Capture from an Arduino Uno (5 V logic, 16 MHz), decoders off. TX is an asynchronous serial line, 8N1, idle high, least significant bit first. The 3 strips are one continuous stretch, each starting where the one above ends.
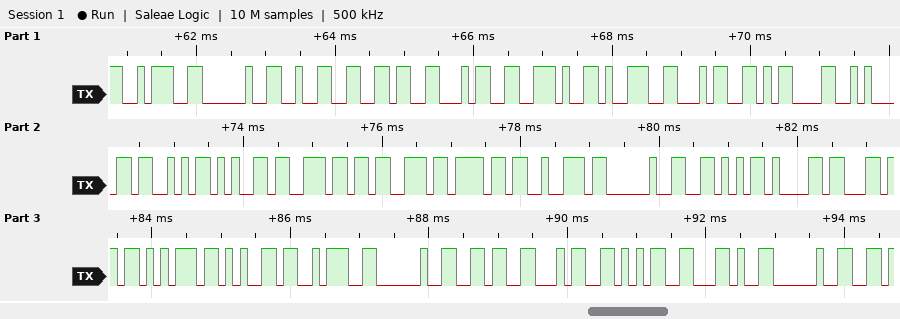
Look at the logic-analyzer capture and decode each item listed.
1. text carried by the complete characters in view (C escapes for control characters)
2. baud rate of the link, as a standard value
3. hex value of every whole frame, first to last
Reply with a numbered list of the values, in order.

1. ": 264.94\r\nSensor Value: 645, "
2. 9600 baud
3. 0x3A 0x20 0x32 0x36 0x34 0x2E 0x39 0x34 0x0D 0x0A 0x53 0x65 0x6E 0x73 0x6F 0x72 0x20 0x56 0x61 0x6C 0x75 0x65 0x3A 0x20 0x36 0x34 0x35 0x2C 0x20
